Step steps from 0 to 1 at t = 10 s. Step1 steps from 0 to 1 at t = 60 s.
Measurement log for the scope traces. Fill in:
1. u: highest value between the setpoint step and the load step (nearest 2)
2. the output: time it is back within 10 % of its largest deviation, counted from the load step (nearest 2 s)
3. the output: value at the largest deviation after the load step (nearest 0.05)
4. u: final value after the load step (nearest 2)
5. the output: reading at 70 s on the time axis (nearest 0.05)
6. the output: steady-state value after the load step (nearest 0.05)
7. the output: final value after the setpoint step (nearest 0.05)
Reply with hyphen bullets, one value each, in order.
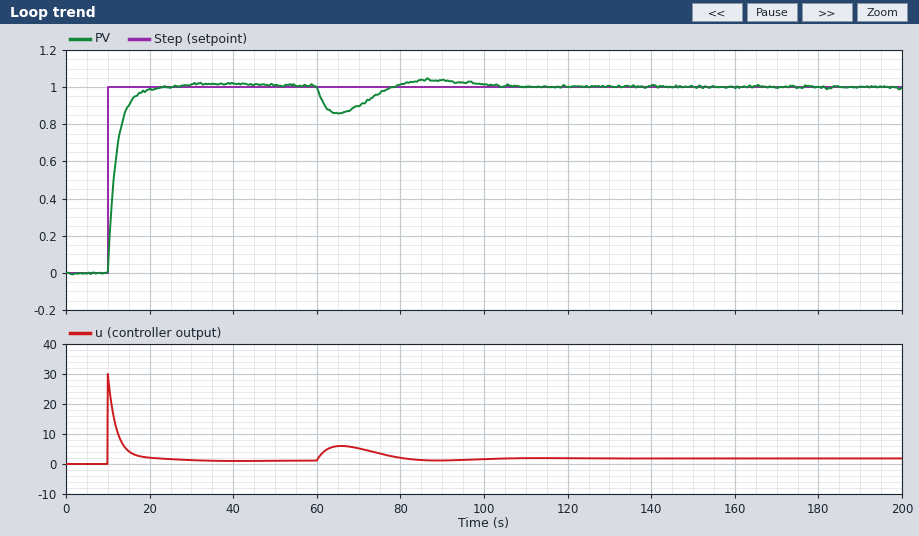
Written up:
- 30
- 40 s
- 0.85
- 2
- 0.90
- 1.00
- 1.00
